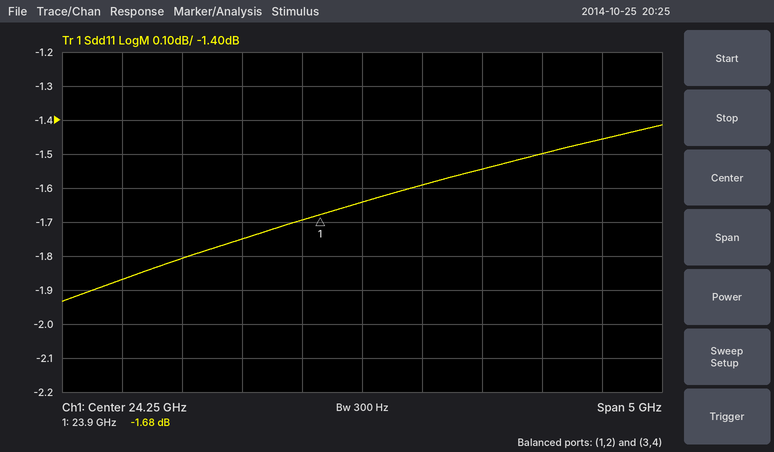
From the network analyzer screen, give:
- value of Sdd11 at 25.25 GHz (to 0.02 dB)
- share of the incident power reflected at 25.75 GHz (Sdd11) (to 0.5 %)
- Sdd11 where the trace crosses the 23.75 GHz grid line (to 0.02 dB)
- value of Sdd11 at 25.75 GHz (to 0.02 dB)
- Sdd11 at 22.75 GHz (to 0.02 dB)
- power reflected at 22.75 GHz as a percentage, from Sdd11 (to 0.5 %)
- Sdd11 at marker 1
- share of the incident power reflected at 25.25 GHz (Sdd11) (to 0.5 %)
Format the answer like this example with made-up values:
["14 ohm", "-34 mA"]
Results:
["-1.54 dB", "71.0 %", "-1.70 dB", "-1.50 dB", "-1.80 dB", "66.0 %", "-1.68 dB", "70.0 %"]
